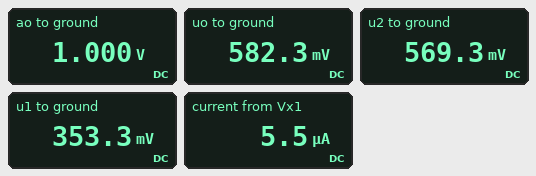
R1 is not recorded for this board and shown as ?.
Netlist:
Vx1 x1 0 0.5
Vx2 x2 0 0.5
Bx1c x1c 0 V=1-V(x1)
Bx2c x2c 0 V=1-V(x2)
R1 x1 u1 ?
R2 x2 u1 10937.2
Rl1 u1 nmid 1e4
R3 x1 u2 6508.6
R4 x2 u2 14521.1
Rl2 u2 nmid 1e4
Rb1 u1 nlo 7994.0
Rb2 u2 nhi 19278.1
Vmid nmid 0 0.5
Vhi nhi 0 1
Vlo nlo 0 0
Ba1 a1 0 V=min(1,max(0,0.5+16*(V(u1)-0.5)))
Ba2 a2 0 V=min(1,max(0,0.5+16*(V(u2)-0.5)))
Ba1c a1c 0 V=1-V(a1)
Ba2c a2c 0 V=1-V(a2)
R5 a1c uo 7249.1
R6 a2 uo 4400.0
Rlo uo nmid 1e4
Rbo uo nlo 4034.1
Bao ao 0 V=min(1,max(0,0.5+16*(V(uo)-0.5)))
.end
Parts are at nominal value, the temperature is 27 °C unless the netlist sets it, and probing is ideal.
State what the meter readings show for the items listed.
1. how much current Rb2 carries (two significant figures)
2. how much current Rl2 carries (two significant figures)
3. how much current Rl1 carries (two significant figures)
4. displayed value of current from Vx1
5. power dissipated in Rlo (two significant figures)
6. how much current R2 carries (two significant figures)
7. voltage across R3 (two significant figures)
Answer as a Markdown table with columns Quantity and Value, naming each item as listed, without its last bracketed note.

| Quantity | Value |
|---|---|
| how much current Rb2 carries | 22 µA |
| how much current Rl2 carries | 6.9 µA |
| how much current Rl1 carries | 15 µA |
| displayed value of current from Vx1 | 5.5 µA |
| power dissipated in Rlo | 680 nW |
| how much current R2 carries | 13 µA |
| voltage across R3 | 69 mV |
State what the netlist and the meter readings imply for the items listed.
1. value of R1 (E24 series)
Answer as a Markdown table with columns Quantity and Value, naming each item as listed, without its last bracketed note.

| Quantity | Value |
|---|---|
| value of R1 | 9.1 kΩ |
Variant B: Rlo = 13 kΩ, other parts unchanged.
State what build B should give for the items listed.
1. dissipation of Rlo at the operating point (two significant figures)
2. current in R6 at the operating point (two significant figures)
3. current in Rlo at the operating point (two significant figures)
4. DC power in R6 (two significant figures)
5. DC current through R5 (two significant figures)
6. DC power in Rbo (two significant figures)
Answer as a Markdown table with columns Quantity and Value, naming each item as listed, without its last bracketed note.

| Quantity | Value |
|---|---|
| dissipation of Rlo at the operating point | 560 nW |
| current in R6 at the operating point | 94 µA |
| current in Rlo at the operating point | 6.5 µA |
| DC power in R6 | 39 µW |
| DC current through R5 | 57 µA |
| DC power in Rbo | 85 µW |
